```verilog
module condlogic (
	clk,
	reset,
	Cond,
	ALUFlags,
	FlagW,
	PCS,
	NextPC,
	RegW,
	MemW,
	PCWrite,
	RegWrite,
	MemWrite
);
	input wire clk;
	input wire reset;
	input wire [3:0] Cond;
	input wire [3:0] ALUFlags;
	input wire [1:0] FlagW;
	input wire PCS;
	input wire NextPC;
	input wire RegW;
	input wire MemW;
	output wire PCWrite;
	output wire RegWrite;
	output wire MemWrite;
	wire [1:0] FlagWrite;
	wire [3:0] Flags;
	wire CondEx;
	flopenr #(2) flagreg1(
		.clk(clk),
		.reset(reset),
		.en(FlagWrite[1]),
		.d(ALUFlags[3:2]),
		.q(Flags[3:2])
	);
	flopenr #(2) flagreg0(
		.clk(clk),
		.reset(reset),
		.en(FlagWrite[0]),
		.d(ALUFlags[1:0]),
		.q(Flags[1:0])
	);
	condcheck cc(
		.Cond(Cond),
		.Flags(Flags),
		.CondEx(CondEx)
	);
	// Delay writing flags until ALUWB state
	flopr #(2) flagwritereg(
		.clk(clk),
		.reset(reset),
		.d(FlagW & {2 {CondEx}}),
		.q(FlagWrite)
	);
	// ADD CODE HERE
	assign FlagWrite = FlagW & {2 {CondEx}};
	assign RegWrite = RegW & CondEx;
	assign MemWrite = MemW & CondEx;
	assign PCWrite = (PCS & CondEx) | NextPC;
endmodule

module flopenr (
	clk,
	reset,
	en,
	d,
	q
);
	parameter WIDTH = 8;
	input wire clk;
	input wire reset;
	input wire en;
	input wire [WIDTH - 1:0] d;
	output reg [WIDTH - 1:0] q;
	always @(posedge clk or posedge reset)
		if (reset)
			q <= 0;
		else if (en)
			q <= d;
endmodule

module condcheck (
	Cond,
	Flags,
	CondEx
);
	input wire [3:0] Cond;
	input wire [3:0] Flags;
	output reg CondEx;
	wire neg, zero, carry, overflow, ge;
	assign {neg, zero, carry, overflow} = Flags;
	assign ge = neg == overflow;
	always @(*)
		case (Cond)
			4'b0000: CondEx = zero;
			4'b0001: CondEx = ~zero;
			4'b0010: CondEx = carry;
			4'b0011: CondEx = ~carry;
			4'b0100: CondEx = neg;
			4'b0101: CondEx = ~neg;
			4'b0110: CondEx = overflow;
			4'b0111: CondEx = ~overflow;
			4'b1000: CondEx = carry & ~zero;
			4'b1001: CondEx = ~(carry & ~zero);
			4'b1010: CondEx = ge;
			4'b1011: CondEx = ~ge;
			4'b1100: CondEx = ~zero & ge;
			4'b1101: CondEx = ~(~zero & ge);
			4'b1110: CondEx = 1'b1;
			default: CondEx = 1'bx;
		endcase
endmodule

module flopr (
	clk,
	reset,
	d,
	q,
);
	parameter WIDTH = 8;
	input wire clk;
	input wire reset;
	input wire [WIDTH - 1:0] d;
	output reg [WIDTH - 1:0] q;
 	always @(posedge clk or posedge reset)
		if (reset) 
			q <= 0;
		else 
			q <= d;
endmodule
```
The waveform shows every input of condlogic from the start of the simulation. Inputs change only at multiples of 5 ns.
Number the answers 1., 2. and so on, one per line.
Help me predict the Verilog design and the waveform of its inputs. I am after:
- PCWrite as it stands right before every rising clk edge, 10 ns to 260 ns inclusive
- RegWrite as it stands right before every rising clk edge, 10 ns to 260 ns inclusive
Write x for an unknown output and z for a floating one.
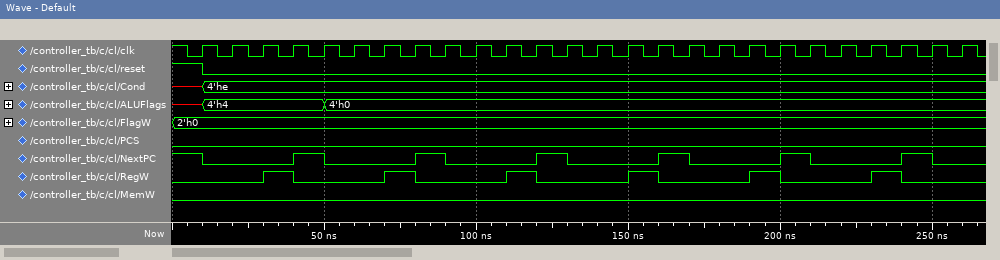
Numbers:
1. 1 0 0 0 1 0 0 0 1 0 0 0 1 0 0 0 1 0 0 0 1 0 0 0 1 0
2. 0 0 0 1 0 0 0 1 0 0 0 1 0 0 0 1 0 0 0 1 0 0 0 1 0 0
